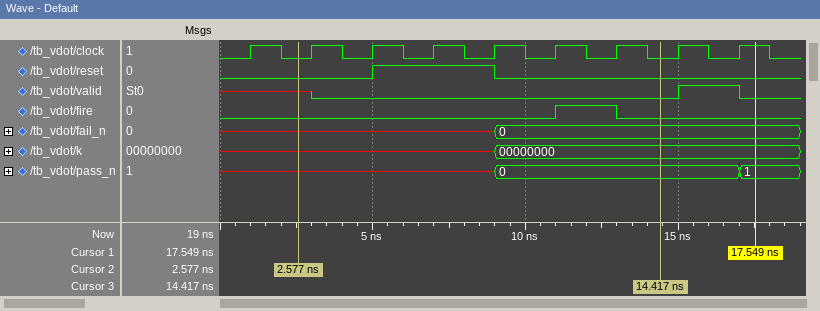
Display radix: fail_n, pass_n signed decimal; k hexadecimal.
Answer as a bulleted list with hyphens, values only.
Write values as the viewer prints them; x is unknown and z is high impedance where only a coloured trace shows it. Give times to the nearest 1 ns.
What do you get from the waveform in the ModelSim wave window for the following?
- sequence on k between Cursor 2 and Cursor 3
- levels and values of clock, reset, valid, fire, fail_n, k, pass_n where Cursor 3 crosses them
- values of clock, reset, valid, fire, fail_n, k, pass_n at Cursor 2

- x, 00000000
- clock=0, reset=0, valid=0, fire=0, fail_n=0, k=00000000, pass_n=0
- clock=0, reset=0, valid=x, fire=0, fail_n=x, k=x, pass_n=x
